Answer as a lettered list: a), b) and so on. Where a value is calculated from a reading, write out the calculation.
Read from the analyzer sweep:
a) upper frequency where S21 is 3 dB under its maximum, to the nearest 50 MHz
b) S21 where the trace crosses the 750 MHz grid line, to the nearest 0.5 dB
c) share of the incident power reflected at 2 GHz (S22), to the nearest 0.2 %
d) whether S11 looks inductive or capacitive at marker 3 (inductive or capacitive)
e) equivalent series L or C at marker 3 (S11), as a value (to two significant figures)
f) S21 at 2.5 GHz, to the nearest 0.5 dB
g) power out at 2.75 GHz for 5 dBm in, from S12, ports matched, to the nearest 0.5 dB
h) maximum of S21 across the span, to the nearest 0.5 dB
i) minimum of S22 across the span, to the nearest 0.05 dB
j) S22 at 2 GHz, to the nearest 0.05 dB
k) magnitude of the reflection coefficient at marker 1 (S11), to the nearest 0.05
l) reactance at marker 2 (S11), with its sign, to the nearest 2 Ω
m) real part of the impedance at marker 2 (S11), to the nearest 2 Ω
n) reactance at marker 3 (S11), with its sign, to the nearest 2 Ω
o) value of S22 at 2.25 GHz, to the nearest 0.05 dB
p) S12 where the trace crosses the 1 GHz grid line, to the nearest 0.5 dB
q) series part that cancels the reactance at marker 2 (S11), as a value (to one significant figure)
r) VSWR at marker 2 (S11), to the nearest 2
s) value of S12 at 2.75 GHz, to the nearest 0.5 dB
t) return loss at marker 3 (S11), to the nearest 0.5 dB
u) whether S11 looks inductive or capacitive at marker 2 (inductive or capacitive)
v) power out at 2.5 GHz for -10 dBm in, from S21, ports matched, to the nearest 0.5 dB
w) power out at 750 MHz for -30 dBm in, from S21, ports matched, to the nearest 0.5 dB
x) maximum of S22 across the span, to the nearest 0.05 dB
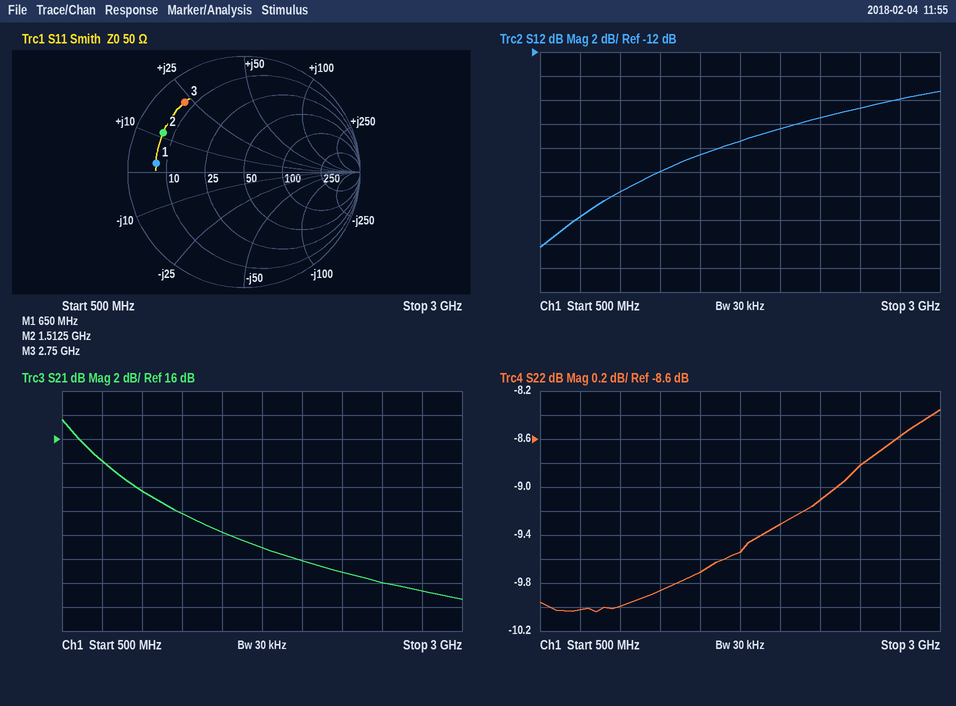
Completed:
a) 700 MHz
b) 14.0 dB
c) 10^(-9.3/10) ≈ 11.7 %, so 11.8 % to the nearest 0.2 %
d) inductive
e) L = 22 Ω/(2π × 2.75 GHz) ≈ 1.3 nH
f) 4.0 dB
g) 5 dBm + (-16.0 dB) = -11.0 dBm
h) 17.5 dB
i) -10.05 dB
j) -9.30 dB
k) 0.75
l) +12 Ω
m) 6 Ω
n) +22 Ω
o) -9.10 dB
p) -23.5 dB
q) C = 1/(2π × 1.5125 GHz × 12 Ω) ≈ 9 pF
r) 8
s) -16.0 dB
t) 2.0 dB
u) inductive
v) -10 dBm + (4.0 dB) = -6.0 dBm
w) -30 dBm + (14.0 dB) = -16.0 dBm
x) -8.35 dB
